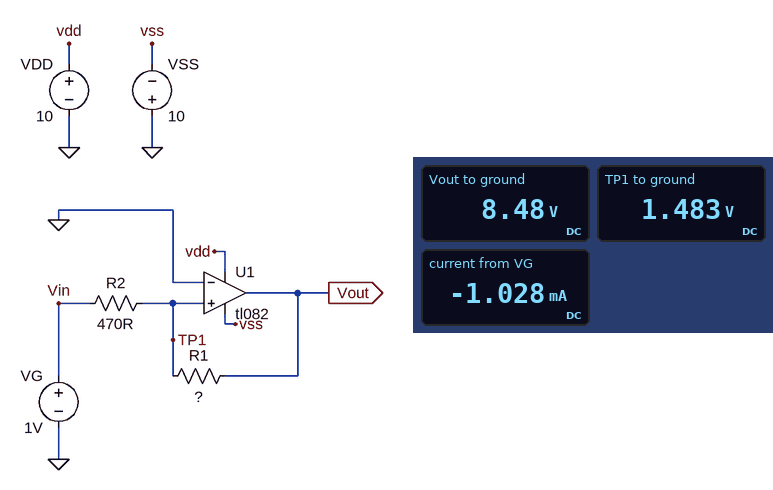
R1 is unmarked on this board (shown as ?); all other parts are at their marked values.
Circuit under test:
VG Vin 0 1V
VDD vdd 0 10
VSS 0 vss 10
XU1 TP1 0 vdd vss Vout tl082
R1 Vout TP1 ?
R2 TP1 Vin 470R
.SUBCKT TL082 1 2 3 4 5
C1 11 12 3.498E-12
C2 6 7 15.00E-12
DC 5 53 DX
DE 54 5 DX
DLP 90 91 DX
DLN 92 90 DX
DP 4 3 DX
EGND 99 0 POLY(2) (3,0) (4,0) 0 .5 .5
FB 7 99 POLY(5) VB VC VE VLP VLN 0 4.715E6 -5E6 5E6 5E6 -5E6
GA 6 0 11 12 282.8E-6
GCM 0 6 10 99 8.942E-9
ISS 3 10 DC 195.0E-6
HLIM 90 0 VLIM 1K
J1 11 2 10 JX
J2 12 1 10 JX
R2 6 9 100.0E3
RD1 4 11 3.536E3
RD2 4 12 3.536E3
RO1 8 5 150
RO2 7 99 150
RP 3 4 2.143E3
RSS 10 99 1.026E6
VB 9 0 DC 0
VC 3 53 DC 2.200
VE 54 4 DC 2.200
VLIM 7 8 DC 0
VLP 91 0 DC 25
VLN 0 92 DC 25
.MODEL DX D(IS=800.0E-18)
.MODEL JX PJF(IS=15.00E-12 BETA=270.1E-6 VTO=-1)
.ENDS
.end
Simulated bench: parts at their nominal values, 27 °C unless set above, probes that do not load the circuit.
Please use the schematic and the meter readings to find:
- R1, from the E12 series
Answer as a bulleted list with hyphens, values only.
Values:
- 6.8 kΩ
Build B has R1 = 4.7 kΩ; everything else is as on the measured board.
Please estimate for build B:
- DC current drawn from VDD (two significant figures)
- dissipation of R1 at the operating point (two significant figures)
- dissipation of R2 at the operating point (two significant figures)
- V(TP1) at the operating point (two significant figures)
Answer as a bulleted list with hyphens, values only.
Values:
- 9.3 mA
- 9.8 mW
- 980 µW
- 1.7 V
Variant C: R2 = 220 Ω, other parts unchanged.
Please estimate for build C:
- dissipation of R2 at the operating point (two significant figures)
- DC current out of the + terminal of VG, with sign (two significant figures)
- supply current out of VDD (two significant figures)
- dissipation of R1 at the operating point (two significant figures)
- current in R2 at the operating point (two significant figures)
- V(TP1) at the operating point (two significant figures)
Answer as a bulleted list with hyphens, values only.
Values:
- 250 µW
- -1.1 mA
- 9.3 mA
- 7.7 mW
- 1.1 mA
- 1.2 V
